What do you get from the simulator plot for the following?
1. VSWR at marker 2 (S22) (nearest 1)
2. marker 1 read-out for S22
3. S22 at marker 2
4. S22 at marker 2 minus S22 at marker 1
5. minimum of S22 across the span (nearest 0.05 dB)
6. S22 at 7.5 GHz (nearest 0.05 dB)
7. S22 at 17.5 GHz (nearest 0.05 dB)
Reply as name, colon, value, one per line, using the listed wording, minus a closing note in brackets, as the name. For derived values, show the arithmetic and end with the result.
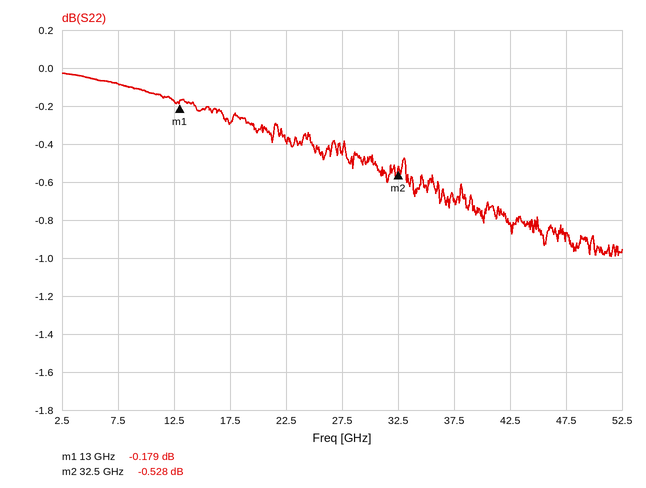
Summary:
VSWR at marker 2 (S22): (1 + 0.9410)/(1 − 0.9410) ≈ 33
marker 1 read-out for S22: -0.179 dB
S22 at marker 2: -0.528 dB
S22 at marker 2 minus S22 at marker 1: -0.528 − (-0.179) = -0.349 dB
minimum of S22 across the span: -1.00 dB
S22 at 7.5 GHz: -0.10 dB
S22 at 17.5 GHz: -0.30 dB
